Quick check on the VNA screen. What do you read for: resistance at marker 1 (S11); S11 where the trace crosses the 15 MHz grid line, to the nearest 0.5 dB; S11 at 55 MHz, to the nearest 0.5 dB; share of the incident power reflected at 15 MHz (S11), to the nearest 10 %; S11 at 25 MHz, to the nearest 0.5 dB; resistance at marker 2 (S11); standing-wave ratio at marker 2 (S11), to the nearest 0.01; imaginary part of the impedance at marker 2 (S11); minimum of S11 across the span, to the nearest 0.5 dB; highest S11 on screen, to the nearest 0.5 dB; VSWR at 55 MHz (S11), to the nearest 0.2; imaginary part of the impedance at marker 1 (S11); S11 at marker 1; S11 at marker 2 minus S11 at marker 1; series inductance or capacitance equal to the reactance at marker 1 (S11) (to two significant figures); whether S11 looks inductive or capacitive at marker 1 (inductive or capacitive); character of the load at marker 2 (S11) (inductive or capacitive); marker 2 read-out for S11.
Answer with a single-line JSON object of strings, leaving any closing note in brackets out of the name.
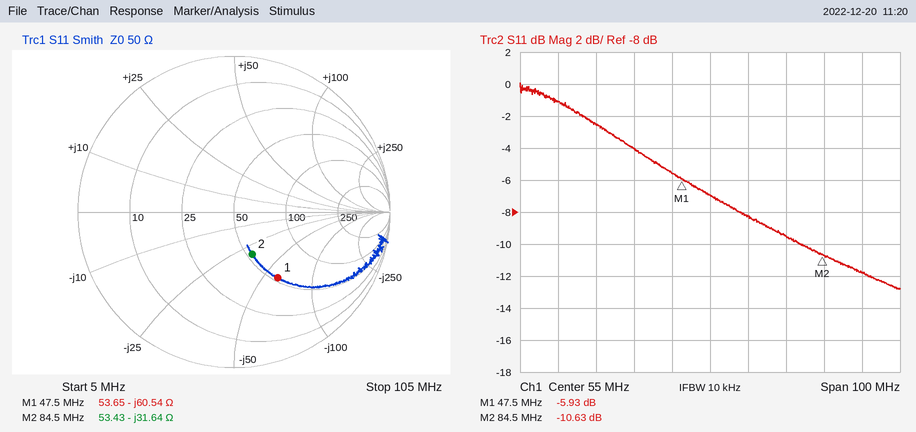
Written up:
{"resistance at marker 1": "53.65 Ω", "S11 where the trace crosses the 15 MHz grid line, to the nearest 0.5 dB": "-1.0 dB", "S11 at 55 MHz, to the nearest 0.5 dB": "-7.0 dB", "share of the incident power reflected at 15 MHz (S11), to the nearest 10 %": "80 %", "S11 at 25 MHz, to the nearest 0.5 dB": "-2.5 dB", "resistance at marker 2": "53.43 Ω", "standing-wave ratio at marker 2 (S11), to the nearest 0.01": "1.83", "imaginary part of the impedance at marker 2": "-31.64 Ω", "minimum of S11 across the span, to the nearest 0.5 dB": "-13.0 dB", "highest S11 on screen, to the nearest 0.5 dB": "0.0 dB", "VSWR at 55 MHz (S11), to the nearest 0.2": "2.6", "imaginary part of the impedance at marker 1": "-60.54 Ω", "S11 at marker 1": "-5.93 dB", "S11 at marker 2 minus S11 at marker 1": "-4.70 dB", "series inductance or capacitance equal to the reactance at marker 1 (S11)": "55 pF", "whether S11 looks inductive or capacitive at marker 1": "capacitive", "character of the load at marker 2 (S11)": "capacitive", "marker 2 read-out for S11": "-10.63 dB"}
